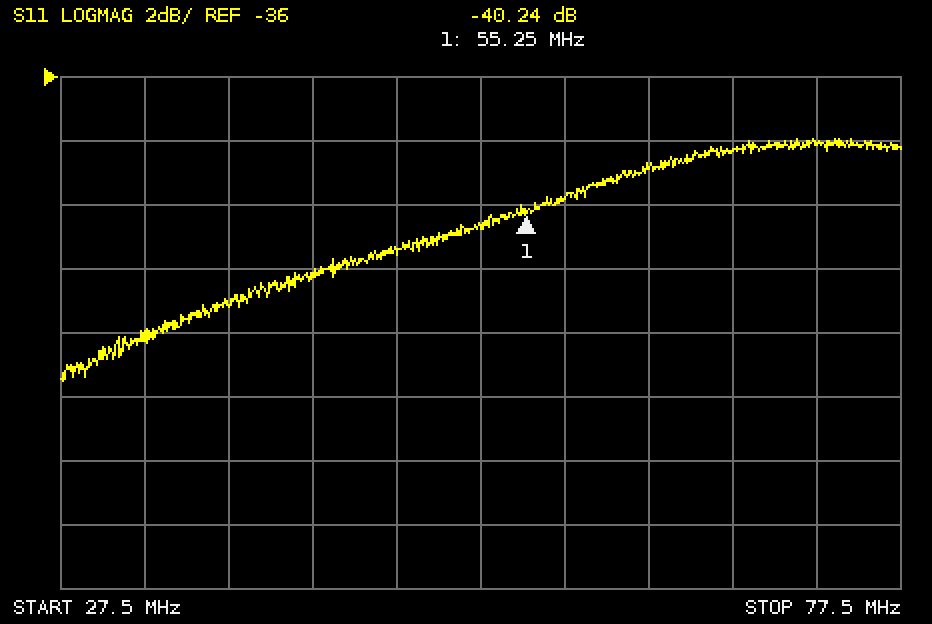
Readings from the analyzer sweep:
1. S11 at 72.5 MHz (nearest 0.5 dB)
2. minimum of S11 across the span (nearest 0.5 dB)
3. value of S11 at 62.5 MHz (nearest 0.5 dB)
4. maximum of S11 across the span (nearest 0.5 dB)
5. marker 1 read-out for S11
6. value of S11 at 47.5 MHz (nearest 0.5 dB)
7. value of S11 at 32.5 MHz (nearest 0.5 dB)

-38.0 dB
-45.5 dB
-39.0 dB
-38.0 dB
-40.24 dB
-41.5 dB
-44.0 dB
